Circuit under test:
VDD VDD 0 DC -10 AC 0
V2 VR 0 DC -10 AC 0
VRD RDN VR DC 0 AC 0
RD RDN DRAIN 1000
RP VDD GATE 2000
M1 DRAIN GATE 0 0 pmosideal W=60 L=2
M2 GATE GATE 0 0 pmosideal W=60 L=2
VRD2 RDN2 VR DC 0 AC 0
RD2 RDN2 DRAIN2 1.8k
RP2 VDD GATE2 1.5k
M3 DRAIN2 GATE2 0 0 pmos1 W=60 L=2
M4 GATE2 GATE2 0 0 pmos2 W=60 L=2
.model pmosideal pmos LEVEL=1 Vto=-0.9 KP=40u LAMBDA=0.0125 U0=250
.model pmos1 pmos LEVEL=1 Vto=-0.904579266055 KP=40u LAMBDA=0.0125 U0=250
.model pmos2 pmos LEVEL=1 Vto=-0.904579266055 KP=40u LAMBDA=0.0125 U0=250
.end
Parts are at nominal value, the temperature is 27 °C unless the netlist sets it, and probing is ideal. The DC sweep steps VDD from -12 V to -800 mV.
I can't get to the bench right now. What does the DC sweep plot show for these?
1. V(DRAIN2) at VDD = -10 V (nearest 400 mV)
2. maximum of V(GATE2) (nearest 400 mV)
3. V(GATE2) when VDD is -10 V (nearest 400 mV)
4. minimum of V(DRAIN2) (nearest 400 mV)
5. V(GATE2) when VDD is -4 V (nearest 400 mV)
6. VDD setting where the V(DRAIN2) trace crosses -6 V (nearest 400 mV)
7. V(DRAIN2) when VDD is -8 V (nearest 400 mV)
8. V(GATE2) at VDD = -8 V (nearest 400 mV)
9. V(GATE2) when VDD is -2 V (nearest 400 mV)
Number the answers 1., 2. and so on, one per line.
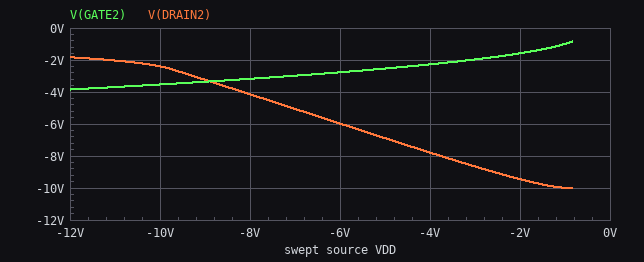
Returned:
1. -2.4 V
2. -800 mV
3. -3.6 V
4. -10.0 V
5. -2.4 V
6. -6.0 V
7. -4.0 V
8. -3.2 V
9. -1.6 V
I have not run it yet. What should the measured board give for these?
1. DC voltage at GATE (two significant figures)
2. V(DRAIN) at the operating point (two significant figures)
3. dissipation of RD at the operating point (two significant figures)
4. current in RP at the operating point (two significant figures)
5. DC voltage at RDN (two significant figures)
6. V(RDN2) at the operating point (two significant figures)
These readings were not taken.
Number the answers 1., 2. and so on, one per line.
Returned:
1. -3.2 V
2. -6.5 V
3. 12 mW
4. 3.4 mA
5. -10 V
6. -10 V
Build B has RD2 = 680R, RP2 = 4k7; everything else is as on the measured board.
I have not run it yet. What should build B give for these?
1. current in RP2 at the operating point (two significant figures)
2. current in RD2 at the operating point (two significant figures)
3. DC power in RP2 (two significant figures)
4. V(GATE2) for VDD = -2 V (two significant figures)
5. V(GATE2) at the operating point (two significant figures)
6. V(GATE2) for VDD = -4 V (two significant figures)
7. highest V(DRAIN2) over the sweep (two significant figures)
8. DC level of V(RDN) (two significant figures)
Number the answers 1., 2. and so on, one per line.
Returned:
1. 1.6 mA
2. 1.7 mA
3. 12 mW
4. -1.4 V
5. -2.5 V
6. -1.8 V
7. -8.6 V
8. -10 V
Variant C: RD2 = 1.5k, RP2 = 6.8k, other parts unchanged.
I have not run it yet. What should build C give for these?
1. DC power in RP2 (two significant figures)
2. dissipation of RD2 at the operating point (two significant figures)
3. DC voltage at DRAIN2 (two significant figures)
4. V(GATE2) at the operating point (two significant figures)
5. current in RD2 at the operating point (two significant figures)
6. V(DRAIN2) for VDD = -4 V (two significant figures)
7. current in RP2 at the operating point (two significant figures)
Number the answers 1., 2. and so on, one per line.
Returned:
1. 8.8 mW
2. 2.2 mW
3. -8.2 V
4. -2.3 V
5. 1.2 mA
6. -9.4 V
7. 1.1 mA
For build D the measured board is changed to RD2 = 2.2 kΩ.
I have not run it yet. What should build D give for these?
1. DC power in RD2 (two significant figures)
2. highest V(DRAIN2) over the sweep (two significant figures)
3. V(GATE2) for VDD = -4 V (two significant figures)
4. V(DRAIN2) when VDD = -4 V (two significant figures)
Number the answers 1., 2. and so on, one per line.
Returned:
1. 31 mW
2. -1.4 V
3. -2.3 V
4. -7.3 V
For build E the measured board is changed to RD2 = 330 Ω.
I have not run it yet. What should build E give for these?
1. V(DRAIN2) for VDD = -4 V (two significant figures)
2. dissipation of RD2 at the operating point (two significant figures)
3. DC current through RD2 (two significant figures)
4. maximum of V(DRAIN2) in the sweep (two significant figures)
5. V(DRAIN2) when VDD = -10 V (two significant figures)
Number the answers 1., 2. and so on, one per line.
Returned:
1. -9.6 V
2. 6.9 mW
3. 4.6 mA
4. -8.1 V
5. -8.5 V
